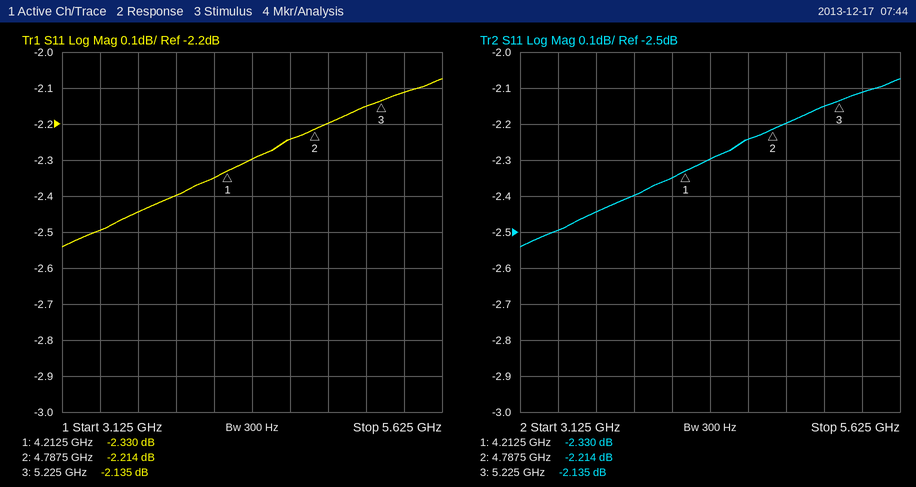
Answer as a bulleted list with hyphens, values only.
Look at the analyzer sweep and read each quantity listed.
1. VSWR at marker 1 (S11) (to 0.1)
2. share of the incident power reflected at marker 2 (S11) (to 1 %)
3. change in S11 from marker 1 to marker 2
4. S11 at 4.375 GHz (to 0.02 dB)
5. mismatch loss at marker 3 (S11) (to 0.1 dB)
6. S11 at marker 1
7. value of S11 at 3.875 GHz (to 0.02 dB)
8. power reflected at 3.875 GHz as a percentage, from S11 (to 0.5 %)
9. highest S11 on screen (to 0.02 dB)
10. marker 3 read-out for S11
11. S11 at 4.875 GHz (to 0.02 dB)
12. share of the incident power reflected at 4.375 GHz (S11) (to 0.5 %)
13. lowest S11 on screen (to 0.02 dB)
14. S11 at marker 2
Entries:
- 7.5
- 60 %
- 0.116 dB
- -2.30 dB
- 4.1 dB
- -2.330 dB
- -2.40 dB
- 57.5 %
- -2.08 dB
- -2.135 dB
- -2.20 dB
- 59.0 %
- -2.54 dB
- -2.214 dB
